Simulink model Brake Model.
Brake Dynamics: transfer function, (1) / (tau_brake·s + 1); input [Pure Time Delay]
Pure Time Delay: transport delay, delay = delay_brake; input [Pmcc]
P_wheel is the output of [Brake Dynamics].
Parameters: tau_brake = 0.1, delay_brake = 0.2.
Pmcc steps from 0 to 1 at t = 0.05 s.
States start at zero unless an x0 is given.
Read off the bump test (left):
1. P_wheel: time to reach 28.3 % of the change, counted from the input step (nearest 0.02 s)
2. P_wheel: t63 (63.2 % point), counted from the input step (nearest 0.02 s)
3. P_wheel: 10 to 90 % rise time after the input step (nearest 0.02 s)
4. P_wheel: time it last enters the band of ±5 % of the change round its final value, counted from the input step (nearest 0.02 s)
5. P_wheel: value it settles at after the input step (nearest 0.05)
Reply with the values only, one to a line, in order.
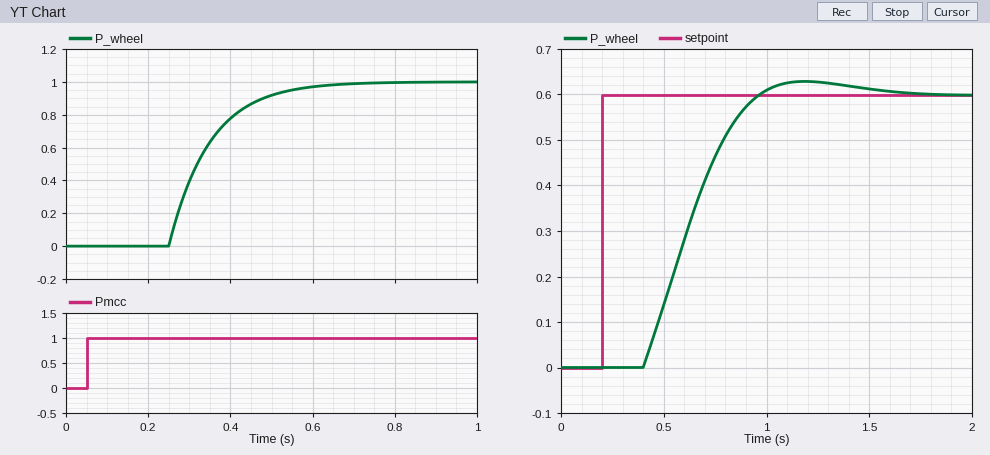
0.24 s
0.30 s
0.22 s
0.50 s
1.00
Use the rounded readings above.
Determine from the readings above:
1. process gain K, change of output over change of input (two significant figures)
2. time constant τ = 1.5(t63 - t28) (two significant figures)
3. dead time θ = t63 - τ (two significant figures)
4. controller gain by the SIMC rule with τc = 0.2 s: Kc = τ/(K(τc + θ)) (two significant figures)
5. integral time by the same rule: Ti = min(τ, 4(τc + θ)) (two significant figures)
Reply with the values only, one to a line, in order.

1.0
0.090 s
0.21 s
0.22
0.090 s
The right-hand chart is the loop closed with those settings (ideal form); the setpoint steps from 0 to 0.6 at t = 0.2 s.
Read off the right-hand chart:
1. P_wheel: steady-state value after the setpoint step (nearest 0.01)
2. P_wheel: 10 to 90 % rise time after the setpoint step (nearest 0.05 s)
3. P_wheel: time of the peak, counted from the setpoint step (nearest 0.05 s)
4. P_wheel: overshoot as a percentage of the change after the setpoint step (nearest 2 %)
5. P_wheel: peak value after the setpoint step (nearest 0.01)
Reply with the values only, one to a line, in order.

0.60
0.40 s
1.00 s
4 %
0.63
